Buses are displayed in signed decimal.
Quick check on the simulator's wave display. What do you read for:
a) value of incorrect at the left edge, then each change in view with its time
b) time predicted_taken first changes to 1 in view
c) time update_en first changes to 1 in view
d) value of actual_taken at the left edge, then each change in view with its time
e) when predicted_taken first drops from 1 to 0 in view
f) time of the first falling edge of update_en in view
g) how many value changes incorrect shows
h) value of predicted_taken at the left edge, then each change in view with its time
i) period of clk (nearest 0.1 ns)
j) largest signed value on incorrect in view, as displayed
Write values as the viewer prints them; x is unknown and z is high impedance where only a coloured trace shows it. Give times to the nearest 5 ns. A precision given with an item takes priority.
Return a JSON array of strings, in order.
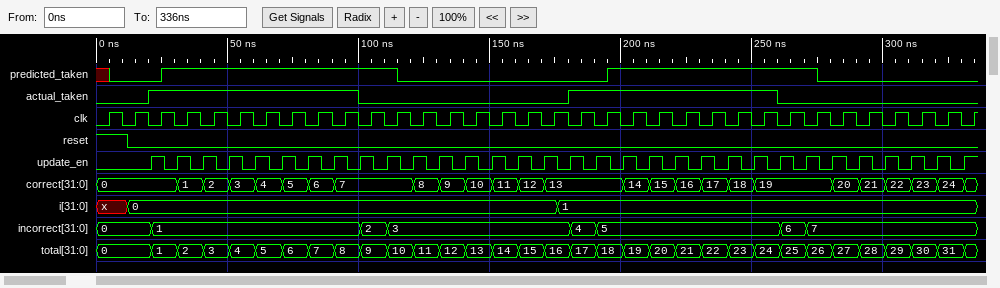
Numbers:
["0, 1 at 20 ns, 2 at 100 ns, 3 at 110 ns, 4 at 180 ns, 5 at 190 ns, 6 at 260 ns, 7 at 270 ns", "25 ns", "20 ns", "0, 1 at 20 ns, 0 at 100 ns, 1 at 180 ns, 0 at 260 ns", "115 ns", "25 ns", "7", "x, 0 at 5 ns, 1 at 25 ns, 0 at 115 ns, 1 at 195 ns, 0 at 275 ns", "10 ns", "7"]
